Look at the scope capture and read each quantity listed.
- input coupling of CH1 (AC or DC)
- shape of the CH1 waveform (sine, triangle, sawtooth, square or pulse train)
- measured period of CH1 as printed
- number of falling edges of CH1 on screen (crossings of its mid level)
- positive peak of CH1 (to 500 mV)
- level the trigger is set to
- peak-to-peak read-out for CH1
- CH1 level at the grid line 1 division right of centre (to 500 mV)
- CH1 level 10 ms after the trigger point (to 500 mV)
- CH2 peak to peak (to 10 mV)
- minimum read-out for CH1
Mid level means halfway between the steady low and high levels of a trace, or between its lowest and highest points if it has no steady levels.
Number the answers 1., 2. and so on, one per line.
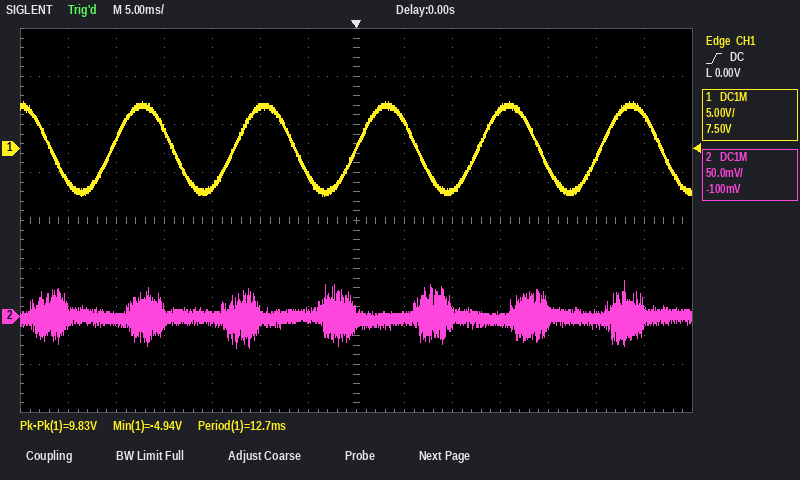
1. DC
2. sine
3. 12.7 ms
4. 6
5. 5.0 V
6. 0.00 V
7. 9.83 V
8. 3.0 V
9. -4.5 V
10. 70 mV
11. -4.94 V
